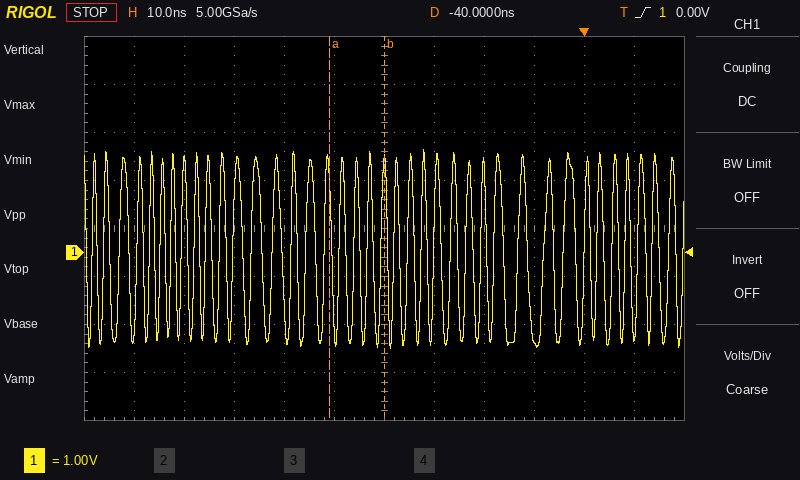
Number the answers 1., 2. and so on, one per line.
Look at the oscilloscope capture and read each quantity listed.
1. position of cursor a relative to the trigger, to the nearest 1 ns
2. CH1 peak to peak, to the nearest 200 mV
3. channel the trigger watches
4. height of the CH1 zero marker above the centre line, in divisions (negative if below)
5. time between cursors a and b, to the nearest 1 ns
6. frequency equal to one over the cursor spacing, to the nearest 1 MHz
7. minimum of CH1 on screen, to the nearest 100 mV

1. -51 ns
2. 4.2 V
3. CH1
4. -0.5 div
5. 11 ns
6. 91 MHz
7. -2.0 V
